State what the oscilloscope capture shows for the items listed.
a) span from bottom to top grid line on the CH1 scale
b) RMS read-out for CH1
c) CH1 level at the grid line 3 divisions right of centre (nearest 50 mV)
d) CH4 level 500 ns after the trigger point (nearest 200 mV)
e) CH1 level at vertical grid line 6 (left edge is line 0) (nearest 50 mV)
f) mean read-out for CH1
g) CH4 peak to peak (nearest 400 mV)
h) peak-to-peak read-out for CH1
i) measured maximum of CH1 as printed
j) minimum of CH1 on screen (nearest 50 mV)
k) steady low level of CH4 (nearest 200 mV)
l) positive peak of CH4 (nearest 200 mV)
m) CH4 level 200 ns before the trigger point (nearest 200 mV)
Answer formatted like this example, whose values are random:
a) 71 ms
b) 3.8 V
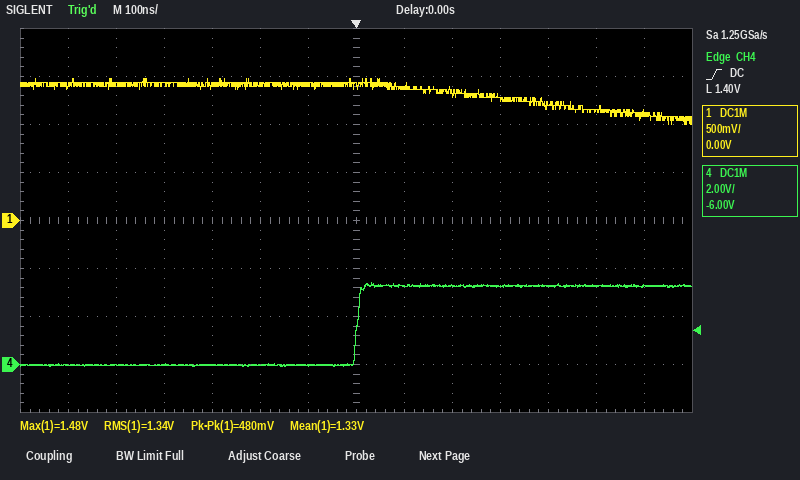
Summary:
a) 4 V
b) 1.34 V
c) 1.25 V
d) 3.2 V
e) 1.40 V
f) 1.33 V
g) 3.6 V
h) 480 mV
i) 1.48 V
j) 1.00 V
k) 0.0 V
l) 3.4 V
m) 0.0 V
